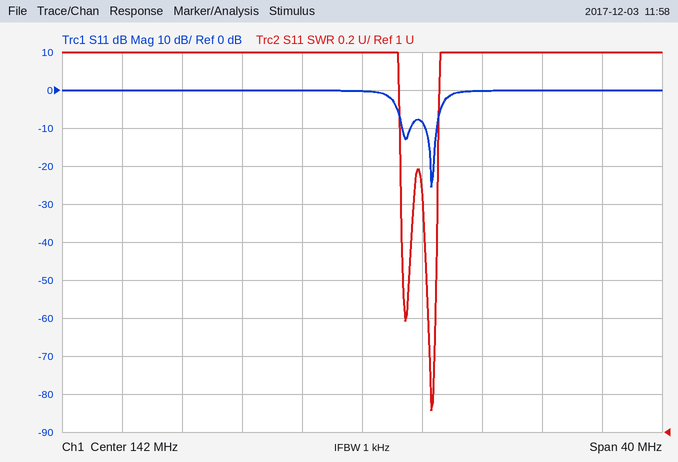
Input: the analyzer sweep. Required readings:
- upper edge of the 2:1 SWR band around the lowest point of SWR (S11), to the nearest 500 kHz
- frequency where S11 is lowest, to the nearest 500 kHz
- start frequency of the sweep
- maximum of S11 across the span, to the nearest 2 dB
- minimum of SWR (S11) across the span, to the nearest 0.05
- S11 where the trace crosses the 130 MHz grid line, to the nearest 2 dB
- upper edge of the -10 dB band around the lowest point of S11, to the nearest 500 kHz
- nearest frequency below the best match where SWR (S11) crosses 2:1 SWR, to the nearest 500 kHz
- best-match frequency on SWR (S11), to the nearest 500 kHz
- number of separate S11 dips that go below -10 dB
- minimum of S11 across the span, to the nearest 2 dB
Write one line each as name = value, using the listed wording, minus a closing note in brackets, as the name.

upper edge of the 2:1 SWR band around the lowest point of SWR (S11), to the nearest 500 kHz = 147.0 MHz
frequency where S11 is lowest, to the nearest 500 kHz = 146.5 MHz
start frequency of the sweep = 122 MHz
maximum of S11 across the span, to the nearest 2 dB = 0 dB
minimum of SWR (S11) across the span, to the nearest 0.05 = 1.10
S11 where the trace crosses the 130 MHz grid line, to the nearest 2 dB = 0 dB
upper edge of the -10 dB band around the lowest point of S11, to the nearest 500 kHz = 147.0 MHz
nearest frequency below the best match where SWR (S11) crosses 2:1 SWR, to the nearest 500 kHz = 146.0 MHz
best-match frequency on SWR (S11), to the nearest 500 kHz = 146.5 MHz
number of separate S11 dips that go below -10 dB = 2
minimum of S11 across the span, to the nearest 2 dB = -26 dB
